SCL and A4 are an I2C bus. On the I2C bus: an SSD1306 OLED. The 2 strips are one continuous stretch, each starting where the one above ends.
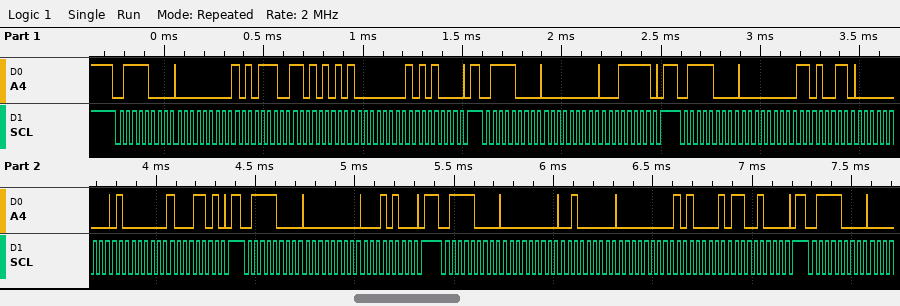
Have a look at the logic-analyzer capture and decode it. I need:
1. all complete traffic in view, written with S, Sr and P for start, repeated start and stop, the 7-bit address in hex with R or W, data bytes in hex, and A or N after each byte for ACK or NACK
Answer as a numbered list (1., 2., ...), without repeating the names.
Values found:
1. S 3CW A 00 A AE A D5 A 80 A A8 A P S 3CW A 00 A 1F A P S 3CW A 00 A D3 A 00 A 40 A 8D A P S 3CW A 00 A 14 A P S 3CW A 00 A 20 A 00 A A1 A C8 A P S 3CW A
